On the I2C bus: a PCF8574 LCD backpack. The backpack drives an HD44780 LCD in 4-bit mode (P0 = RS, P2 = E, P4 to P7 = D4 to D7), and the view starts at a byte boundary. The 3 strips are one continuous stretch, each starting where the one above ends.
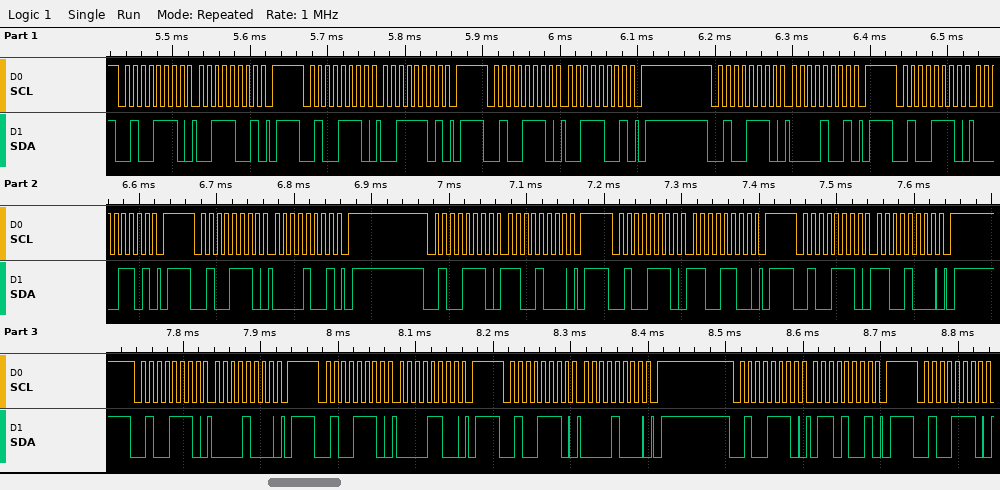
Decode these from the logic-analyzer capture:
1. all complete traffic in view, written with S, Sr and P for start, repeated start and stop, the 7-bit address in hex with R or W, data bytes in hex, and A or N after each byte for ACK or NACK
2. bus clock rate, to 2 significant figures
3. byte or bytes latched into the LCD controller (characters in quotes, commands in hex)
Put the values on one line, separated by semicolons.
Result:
S 27W A 39 A P S 27W A 3D A P S 27W A 39 A P S 27W A 09 A P S 27W A 0D A P S 27W A 09 A P S 27W A C8 A P S 27W A CC A P S 27W A C8 A P S 27W A 08 A P S 27W A 0C A P S 27W A 08 A P S 27W A 69 A P S 27W A; 100 kHz; '0' 0xC0
